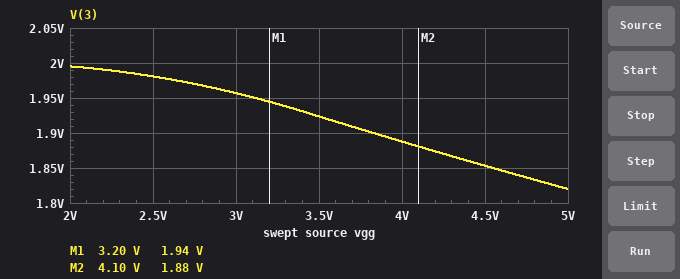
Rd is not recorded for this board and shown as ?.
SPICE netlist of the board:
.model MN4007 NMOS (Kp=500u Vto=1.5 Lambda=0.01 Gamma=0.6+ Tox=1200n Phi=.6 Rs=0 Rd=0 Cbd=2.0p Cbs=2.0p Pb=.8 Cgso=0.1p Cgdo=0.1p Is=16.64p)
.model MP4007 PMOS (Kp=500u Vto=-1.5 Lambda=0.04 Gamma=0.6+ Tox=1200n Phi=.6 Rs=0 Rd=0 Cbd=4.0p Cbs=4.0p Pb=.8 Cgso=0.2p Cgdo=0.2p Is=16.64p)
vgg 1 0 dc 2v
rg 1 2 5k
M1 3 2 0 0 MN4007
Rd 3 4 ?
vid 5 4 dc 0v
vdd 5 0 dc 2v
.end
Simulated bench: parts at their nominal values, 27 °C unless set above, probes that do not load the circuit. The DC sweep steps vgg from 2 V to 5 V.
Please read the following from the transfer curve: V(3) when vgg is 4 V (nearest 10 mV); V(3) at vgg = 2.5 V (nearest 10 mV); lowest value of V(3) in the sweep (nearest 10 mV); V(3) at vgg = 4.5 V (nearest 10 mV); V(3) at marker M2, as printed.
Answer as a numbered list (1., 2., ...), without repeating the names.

1. 1.89 V
2. 1.98 V
3. 1.82 V
4. 1.85 V
5. 1.88 V
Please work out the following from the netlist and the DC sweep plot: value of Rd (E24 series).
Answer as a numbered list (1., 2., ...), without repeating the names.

1. 75 Ω
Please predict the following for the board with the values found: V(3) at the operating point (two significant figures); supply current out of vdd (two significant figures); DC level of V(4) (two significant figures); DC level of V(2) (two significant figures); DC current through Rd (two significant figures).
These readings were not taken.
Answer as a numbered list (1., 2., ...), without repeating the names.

1. 2.0 V
2. 64 µA
3. 2.0 V
4. 2.0 V
5. 64 µA
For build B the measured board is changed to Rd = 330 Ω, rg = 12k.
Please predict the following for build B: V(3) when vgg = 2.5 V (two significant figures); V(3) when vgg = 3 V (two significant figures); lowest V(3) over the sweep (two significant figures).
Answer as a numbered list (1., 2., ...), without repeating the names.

1. 1.9 V
2. 1.8 V
3. 1.4 V
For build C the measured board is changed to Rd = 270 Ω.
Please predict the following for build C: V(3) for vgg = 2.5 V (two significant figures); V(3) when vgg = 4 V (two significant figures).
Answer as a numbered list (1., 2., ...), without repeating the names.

1. 1.9 V
2. 1.6 V
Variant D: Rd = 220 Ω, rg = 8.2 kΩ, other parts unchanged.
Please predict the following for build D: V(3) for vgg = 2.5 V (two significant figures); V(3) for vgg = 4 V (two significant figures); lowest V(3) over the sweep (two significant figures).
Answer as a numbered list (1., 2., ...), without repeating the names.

1. 1.9 V
2. 1.7 V
3. 1.5 V
